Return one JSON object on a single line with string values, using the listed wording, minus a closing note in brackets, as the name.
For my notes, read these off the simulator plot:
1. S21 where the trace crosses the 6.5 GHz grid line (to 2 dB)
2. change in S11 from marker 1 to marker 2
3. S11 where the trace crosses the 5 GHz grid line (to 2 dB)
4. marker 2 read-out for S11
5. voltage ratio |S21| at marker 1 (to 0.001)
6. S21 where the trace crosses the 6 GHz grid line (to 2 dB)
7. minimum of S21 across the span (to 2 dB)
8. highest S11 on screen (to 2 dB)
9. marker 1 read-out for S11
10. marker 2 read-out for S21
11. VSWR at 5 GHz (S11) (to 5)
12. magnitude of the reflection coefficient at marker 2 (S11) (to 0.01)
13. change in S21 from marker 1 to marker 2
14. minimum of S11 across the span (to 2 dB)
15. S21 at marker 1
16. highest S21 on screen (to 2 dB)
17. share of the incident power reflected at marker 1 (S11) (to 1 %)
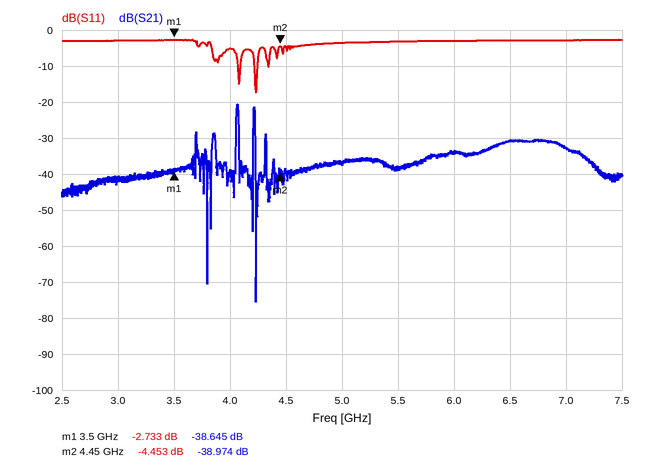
{"S21 where the trace crosses the 6.5 GHz grid line": "-30 dB", "change in S11 from marker 1 to marker 2": "-1.720 dB", "S11 where the trace crosses the 5 GHz grid line": "-4 dB", "marker 2 read-out for S11": "-4.453 dB", "voltage ratio |S21| at marker 1": "0.012", "S21 where the trace crosses the 6 GHz grid line": "-34 dB", "minimum of S21 across the span": "-76 dB", "highest S11 on screen": "-2 dB", "marker 1 read-out for S11": "-2.733 dB", "marker 2 read-out for S21": "-38.974 dB", "VSWR at 5 GHz (S11)": "5", "magnitude of the reflection coefficient at marker 2 (S11)": "0.60", "change in S21 from marker 1 to marker 2": "-0.329 dB", "minimum of S11 across the span": "-18 dB", "S21 at marker 1": "-38.645 dB", "highest S21 on screen": "-20 dB", "share of the incident power reflected at marker 1 (S11)": "53 %"}
